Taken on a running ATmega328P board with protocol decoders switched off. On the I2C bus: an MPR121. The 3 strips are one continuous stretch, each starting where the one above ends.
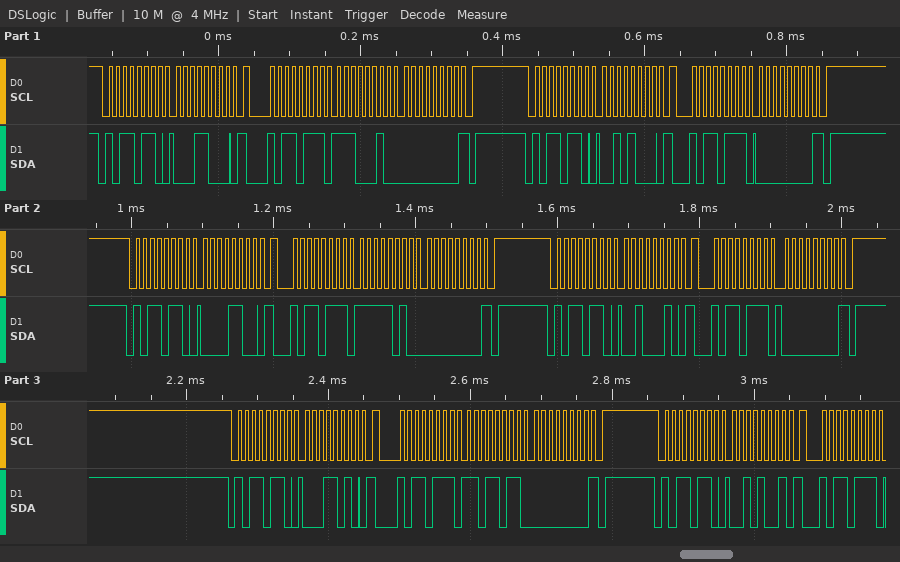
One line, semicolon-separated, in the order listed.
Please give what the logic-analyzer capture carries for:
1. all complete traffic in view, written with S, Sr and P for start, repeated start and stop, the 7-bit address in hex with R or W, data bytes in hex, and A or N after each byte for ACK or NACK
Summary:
S 5BW A 18 A Sr 5BR A E2 A 00 N P S 5BW A 28 A Sr 5BR A 00 N P S 5BW A 0C A Sr 5BR A FA A 00 N P S 5BW A 22 A Sr 5BR A 00 N P S 5BW A 1A A Sr 5BR A DB A 00 N P S 5BW A 29 A Sr 5BR A
